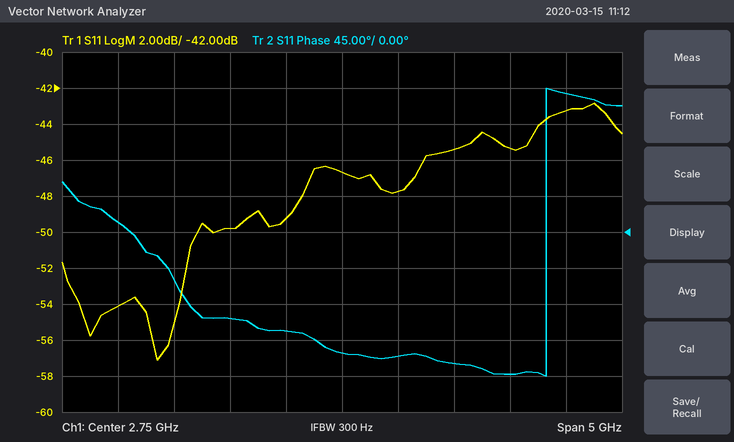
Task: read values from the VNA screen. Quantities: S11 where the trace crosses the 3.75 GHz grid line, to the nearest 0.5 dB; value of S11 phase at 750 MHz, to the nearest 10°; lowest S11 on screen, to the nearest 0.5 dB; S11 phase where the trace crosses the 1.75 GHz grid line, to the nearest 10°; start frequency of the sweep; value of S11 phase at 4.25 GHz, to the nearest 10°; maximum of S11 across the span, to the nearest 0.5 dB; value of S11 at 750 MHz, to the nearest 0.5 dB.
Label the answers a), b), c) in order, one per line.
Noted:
a) -45.5 dB
b) 10°
c) -57.0 dB
d) -110°
e) 250 MHz
f) -180°
g) -43.0 dB
h) -54.0 dB
